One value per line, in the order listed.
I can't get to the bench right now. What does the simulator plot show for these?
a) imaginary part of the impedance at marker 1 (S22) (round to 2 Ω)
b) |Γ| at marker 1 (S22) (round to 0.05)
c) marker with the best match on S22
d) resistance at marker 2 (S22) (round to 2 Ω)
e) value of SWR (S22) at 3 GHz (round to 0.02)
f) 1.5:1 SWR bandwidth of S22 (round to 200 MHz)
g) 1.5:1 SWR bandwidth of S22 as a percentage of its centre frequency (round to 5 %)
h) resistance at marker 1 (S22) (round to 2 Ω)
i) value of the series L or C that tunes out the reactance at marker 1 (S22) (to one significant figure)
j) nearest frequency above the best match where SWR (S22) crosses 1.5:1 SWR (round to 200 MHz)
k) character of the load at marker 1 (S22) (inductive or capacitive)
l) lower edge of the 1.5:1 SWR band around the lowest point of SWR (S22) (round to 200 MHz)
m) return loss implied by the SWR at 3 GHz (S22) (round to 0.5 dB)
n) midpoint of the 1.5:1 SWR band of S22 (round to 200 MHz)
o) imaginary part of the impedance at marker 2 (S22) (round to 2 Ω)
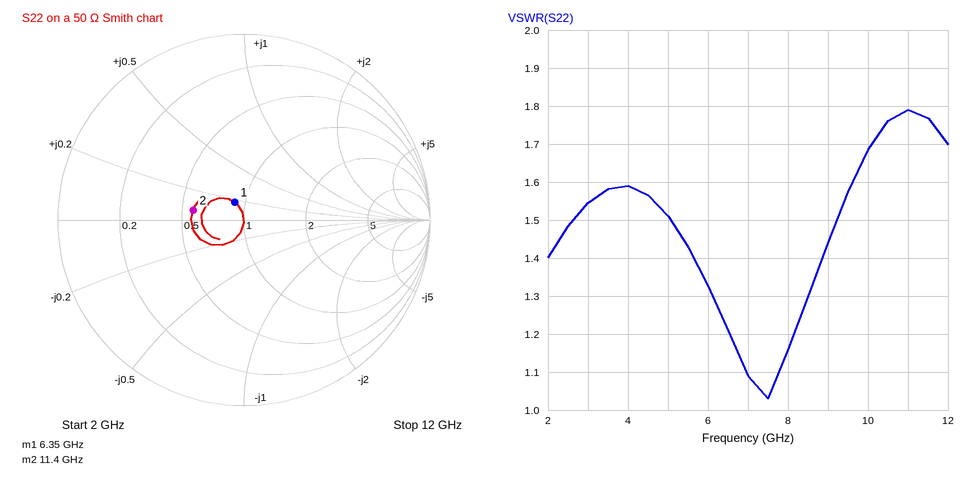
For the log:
+8 Ω
0.10
marker 1
28 Ω
1.54
4.2 GHz
60 %
44 Ω
3 pF
9.2 GHz
inductive
5.0 GHz
13.5 dB
7.2 GHz
+4 Ω
